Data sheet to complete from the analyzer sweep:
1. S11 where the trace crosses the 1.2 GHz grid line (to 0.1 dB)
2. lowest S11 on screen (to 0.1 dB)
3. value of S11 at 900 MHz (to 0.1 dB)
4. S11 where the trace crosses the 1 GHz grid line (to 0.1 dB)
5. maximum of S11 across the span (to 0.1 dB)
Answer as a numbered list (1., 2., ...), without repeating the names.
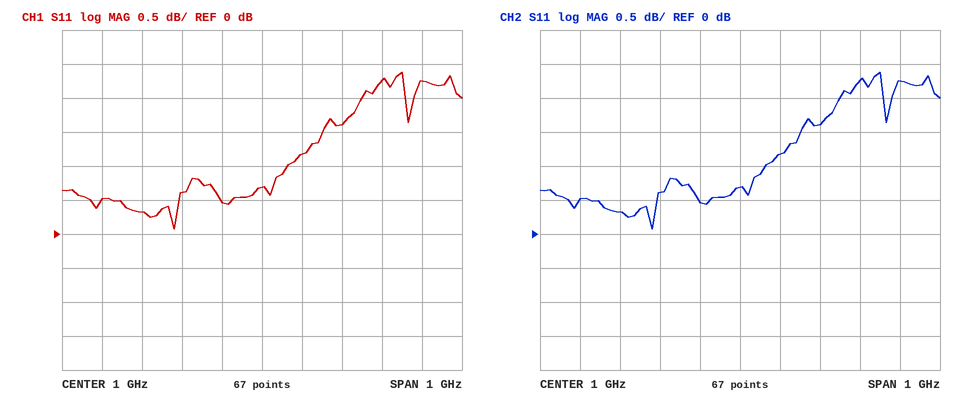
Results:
1. 1.6 dB
2. 0.1 dB
3. 0.5 dB
4. 0.7 dB
5. 2.4 dB
